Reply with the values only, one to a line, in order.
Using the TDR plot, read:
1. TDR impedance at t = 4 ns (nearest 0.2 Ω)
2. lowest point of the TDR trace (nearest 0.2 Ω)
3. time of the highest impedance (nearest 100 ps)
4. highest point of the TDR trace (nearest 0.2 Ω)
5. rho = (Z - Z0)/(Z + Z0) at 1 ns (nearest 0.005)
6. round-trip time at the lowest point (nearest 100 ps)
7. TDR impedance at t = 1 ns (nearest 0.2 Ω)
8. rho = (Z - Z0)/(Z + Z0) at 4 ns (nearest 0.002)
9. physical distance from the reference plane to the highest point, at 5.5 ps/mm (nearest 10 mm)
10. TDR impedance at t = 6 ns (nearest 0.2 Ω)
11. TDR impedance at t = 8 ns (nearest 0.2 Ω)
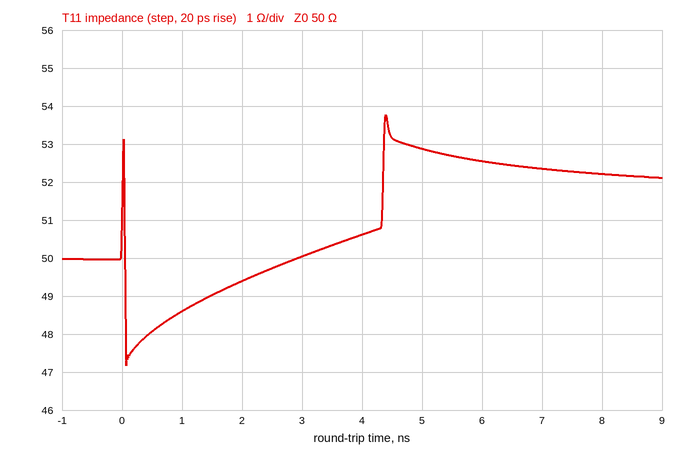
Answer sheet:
50.6 Ω
47.2 Ω
4.4 ns
53.8 Ω
-0.015
100 ps
48.6 Ω
+0.006
400 mm
52.6 Ω
52.2 Ω
